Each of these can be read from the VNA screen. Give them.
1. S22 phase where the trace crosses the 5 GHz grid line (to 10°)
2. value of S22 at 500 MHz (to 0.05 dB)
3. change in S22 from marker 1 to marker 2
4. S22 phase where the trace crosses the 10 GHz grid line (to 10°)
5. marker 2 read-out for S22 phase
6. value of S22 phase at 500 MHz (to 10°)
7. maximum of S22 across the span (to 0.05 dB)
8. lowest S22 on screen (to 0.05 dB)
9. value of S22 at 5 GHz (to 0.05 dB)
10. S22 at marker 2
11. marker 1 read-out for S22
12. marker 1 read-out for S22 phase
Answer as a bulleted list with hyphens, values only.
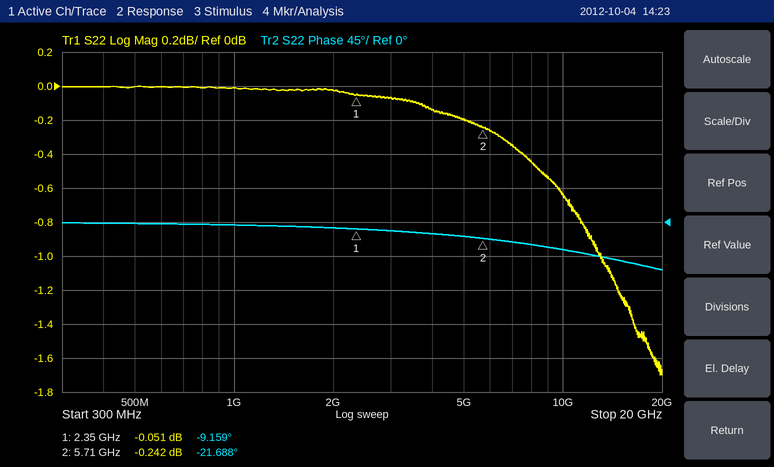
- -20°
- 0.00 dB
- -0.191 dB
- -40°
- -21.688°
- 0°
- 0.00 dB
- -1.70 dB
- -0.20 dB
- -0.242 dB
- -0.051 dB
- -9.159°
